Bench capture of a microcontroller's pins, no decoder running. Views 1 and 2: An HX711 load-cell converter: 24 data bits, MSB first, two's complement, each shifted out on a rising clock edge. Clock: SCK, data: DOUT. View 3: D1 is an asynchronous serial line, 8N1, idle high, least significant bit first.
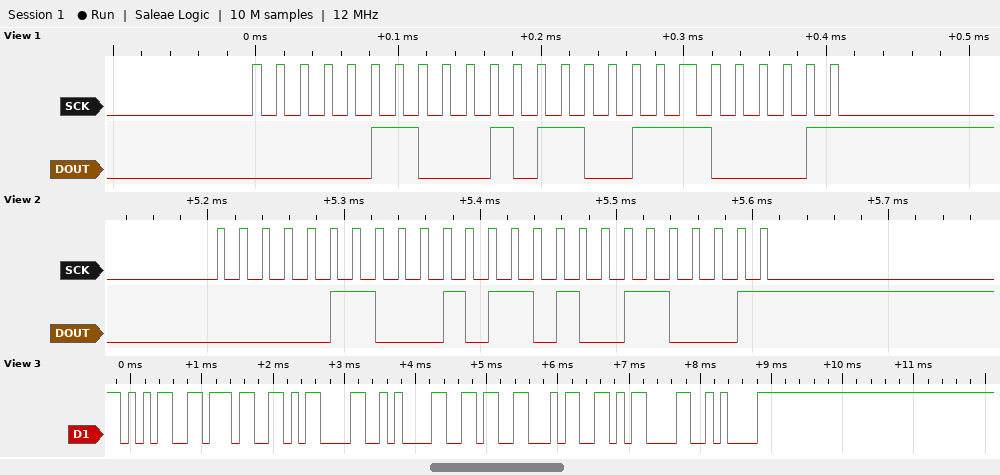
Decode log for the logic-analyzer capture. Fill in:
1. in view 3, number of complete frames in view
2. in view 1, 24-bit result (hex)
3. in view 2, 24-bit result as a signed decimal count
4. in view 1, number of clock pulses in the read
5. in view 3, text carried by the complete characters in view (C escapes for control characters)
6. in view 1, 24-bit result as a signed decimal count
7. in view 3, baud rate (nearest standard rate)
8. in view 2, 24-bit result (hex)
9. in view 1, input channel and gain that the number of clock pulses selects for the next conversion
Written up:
8
0x062CE1
404785
25
"57\r\n64\r\n"
404705
9600 baud
0x062D31
channel A, gain 128
